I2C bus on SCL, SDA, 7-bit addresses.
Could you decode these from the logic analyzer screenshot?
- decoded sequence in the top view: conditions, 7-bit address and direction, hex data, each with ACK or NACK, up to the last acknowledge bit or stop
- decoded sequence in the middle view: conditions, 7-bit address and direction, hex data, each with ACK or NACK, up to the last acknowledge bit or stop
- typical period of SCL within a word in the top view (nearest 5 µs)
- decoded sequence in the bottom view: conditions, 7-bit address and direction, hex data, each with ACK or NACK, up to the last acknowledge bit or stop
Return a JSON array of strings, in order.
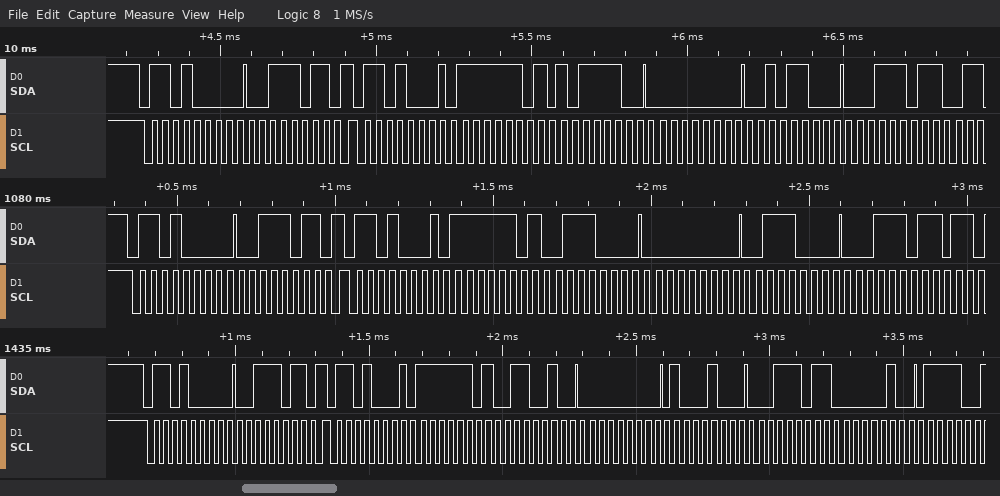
["start, address 68 write ACK, 3B ACK, repeated start, address 68 read ACK, FD ACK, BC ACK, 00 ACK, 58 ACK, 3B ACK", "start, address 68 write ACK, 3B ACK, repeated start, address 68 read ACK, FD ACK, 70 ACK, 00 ACK, 70 ACK, 3B ACK", "35 µs", "start, address 68 write ACK, 3B ACK, repeated start, address 68 read ACK, FD ACK, 64 ACK, 00 ACK, 88 ACK, 3B ACK, 04 ACK"]
